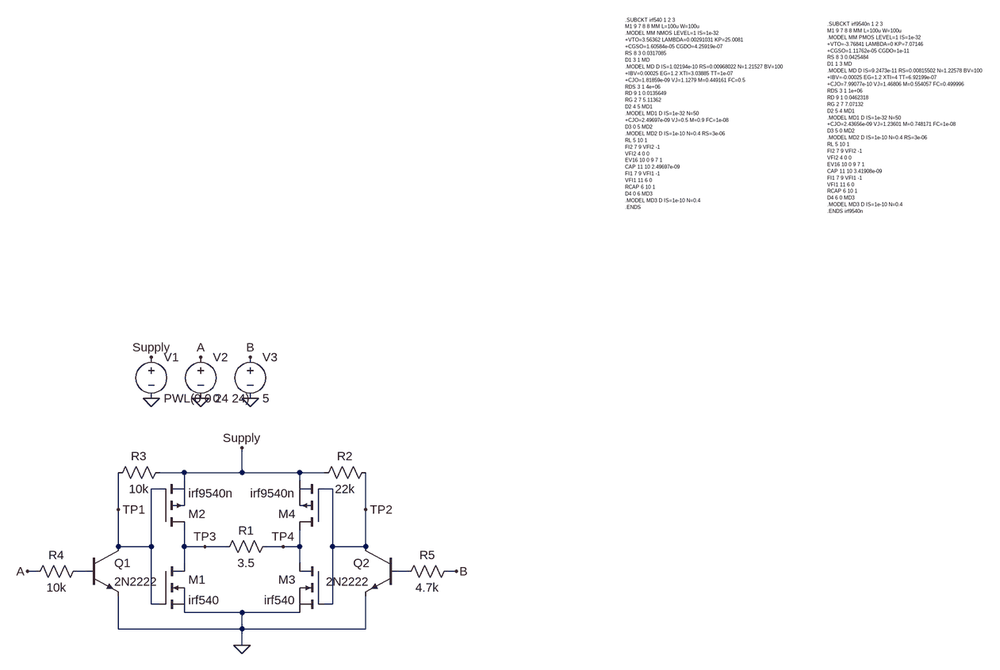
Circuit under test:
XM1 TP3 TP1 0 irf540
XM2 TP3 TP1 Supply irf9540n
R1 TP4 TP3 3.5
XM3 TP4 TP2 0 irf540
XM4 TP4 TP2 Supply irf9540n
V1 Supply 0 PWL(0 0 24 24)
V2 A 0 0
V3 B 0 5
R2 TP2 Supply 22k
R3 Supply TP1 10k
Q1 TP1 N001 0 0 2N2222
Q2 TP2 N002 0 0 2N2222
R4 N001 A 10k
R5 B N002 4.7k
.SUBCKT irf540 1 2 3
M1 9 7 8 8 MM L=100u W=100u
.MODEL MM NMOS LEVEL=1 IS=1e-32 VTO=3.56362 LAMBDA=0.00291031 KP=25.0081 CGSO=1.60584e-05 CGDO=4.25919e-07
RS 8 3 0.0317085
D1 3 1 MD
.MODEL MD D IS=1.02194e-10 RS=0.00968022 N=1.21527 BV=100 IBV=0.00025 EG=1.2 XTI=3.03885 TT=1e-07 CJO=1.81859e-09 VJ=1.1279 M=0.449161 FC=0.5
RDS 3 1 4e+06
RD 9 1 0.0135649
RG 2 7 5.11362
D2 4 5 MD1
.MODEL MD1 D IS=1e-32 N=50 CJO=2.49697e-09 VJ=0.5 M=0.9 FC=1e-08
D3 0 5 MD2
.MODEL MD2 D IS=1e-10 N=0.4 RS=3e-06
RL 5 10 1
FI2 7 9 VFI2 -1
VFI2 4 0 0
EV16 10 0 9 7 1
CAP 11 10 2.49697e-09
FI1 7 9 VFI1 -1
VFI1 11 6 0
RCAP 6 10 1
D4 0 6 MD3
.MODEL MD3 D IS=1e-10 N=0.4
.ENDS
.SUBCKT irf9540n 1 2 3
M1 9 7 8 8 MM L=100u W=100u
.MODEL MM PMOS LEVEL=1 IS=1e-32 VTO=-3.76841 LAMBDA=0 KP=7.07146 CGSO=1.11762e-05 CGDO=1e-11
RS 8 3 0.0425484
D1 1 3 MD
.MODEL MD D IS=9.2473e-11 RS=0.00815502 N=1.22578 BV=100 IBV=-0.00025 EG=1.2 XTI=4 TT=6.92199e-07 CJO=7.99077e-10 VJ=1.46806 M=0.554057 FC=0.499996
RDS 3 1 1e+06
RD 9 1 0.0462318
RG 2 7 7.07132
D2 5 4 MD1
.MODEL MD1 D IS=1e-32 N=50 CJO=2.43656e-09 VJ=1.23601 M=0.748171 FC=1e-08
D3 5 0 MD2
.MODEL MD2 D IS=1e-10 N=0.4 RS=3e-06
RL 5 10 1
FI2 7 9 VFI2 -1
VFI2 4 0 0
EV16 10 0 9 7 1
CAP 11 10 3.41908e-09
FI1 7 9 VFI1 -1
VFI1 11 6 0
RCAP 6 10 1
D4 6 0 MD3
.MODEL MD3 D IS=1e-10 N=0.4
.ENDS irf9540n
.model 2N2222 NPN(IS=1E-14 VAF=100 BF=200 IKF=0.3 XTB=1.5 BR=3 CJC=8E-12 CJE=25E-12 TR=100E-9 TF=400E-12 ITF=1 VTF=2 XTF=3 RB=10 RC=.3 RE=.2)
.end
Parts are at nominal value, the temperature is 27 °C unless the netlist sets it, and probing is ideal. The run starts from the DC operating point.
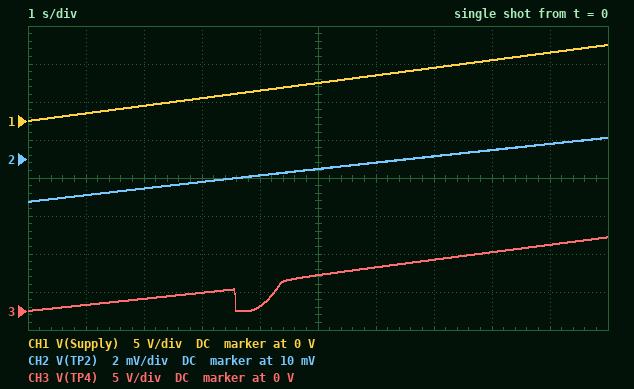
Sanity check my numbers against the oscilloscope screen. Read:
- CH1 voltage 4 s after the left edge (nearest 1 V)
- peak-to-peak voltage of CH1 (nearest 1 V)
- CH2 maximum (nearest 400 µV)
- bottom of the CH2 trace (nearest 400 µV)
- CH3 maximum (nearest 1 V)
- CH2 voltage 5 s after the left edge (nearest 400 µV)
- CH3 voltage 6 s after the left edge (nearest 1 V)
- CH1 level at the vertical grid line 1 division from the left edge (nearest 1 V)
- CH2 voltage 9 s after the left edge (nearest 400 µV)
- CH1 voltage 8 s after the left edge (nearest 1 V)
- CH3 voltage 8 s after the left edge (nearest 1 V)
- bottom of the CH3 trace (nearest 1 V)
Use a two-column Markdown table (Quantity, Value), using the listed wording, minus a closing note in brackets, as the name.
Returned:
| Quantity | Value |
|---|---|
| CH1 voltage 4 s after the left edge | 4 V |
| peak-to-peak voltage of CH1 | 10 V |
| CH2 maximum | 11.2 mV |
| bottom of the CH2 trace | 7.6 mV |
| CH3 maximum | 10 V |
| CH2 voltage 5 s after the left edge | 9.6 mV |
| CH3 voltage 6 s after the left edge | 6 V |
| CH1 level at the vertical grid line 1 division from the left edge | 1 V |
| CH2 voltage 9 s after the left edge | 10.8 mV |
| CH1 voltage 8 s after the left edge | 8 V |
| CH3 voltage 8 s after the left edge | 8 V |
| bottom of the CH3 trace | 0 V |
